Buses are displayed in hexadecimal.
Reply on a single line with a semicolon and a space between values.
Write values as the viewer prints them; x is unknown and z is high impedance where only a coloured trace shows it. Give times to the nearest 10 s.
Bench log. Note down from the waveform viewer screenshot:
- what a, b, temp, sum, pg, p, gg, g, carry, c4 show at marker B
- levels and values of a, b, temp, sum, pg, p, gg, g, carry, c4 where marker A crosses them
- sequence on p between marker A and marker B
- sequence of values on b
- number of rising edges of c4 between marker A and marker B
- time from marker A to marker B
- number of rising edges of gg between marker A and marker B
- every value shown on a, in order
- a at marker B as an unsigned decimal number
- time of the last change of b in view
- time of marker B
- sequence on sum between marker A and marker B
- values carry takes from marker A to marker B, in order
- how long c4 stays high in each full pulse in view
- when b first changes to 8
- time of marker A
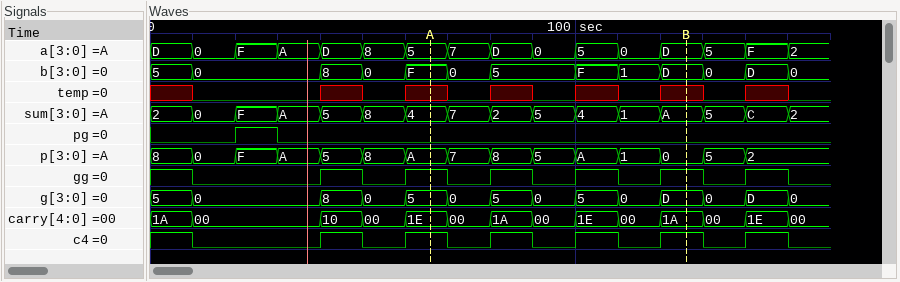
a=D, b=D, temp=x, sum=A, pg=0, p=0, gg=1, g=D, carry=1A, c4=1; a=5, b=F, temp=x, sum=4, pg=0, p=A, gg=1, g=5, carry=1E, c4=1; A, 7, 8, 5, A, 1, 0; 5, 0, 8, 0, F, 0, 5, F, 1, D, 0, D, 0; 3; 60 s; 3; D, 0, F, A, D, 8, 5, 7, D, 0, 5, 0, D, 5, F, 2; 13; 150 s; 130 s; 4, 7, 2, 5, 4, 1, A; 1E, 00, 1A, 00, 1E, 00, 1A; 10 s, 10 s, 10 s, 10 s, 10 s, 10 s; 40 s; 70 s
